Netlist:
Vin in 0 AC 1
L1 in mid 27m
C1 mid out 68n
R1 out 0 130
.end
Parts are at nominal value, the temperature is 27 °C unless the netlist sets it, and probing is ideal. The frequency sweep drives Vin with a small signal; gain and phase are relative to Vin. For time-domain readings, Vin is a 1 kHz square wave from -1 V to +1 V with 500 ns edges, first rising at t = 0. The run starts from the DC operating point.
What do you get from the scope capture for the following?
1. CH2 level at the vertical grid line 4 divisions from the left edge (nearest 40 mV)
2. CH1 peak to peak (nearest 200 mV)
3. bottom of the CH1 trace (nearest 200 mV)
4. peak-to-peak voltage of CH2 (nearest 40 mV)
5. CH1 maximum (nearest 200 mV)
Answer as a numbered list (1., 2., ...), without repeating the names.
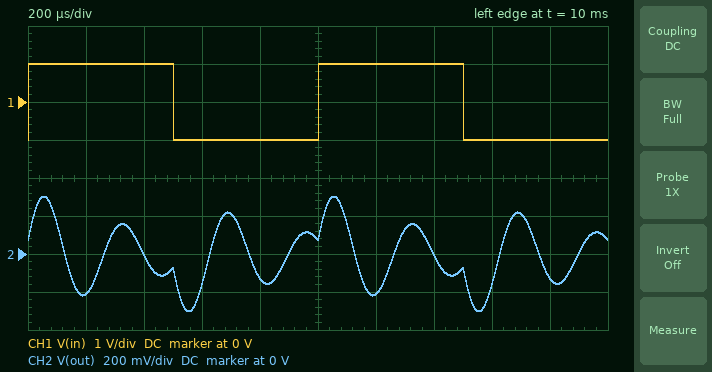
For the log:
1. -120 mV
2. 2.0 V
3. -1.0 V
4. 600 mV
5. 1.0 V
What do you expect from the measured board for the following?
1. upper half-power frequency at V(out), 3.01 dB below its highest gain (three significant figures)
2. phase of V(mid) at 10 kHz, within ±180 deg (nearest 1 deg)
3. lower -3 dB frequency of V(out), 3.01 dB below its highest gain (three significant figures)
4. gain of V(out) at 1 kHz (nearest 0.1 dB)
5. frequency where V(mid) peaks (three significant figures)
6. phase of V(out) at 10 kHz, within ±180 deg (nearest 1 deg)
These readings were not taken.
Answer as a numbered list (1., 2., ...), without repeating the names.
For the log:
1. 4.12 kHz
2. -146 deg
3. 3.35 kHz
4. -24.5 dB
5. 3.68 kHz
6. -85 deg
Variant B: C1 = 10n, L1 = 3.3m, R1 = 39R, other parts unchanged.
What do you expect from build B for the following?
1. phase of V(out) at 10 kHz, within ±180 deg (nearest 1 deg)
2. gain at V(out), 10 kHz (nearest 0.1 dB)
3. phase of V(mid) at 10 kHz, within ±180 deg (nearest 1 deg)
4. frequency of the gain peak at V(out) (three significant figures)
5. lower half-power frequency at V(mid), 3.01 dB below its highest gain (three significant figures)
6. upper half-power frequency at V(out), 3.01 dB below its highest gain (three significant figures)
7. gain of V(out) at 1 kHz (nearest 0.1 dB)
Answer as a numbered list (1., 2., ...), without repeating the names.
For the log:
1. 88 deg
2. -31.0 dB
3. 0 deg
4. 27.7 kHz
5. 26.7 kHz
6. 28.7 kHz
7. -52.2 dB
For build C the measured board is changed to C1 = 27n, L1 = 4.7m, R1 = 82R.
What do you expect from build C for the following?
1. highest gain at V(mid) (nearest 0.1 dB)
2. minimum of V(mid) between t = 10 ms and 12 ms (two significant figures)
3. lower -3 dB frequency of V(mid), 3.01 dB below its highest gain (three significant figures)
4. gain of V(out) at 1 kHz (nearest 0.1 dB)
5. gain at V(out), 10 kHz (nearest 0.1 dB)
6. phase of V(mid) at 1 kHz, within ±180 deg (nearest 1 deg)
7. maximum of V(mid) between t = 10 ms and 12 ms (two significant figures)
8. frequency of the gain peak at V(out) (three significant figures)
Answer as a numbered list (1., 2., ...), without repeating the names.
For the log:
1. 14.3 dB
2. -2.5 V
3. 12.5 kHz
4. -37.1 dB
5. -11.4 dB
6. 0 deg
7. 2.5 V
8. 14.1 kHz
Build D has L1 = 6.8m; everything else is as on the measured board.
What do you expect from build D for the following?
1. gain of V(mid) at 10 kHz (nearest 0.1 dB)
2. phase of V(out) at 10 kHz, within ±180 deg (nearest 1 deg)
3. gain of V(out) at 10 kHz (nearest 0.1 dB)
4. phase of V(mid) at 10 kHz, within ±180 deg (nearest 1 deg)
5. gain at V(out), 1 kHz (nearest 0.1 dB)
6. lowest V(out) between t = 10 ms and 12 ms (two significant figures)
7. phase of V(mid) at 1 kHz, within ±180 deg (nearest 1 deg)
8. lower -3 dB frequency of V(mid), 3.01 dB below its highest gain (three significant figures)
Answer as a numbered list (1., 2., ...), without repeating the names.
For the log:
1. 1.2 dB
2. -56 deg
3. -5.1 dB
4. -117 deg
5. -25.0 dB
6. -620 mV
7. 0 deg
8. 5.42 kHz
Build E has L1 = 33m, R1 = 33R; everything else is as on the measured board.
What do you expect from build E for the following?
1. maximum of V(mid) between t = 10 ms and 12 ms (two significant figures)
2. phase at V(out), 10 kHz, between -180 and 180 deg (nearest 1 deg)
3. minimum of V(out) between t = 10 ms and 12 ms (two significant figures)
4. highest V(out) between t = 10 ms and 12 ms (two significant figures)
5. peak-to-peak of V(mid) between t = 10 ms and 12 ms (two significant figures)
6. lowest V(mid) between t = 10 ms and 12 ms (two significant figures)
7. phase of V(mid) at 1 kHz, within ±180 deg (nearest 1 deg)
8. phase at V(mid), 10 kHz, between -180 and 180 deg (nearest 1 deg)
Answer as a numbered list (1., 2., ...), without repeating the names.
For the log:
1. 3.0 V
2. -89 deg
3. -96 mV
4. 96 mV
5. 5.9 V
6. -3.0 V
7. 0 deg
8. -171 deg
